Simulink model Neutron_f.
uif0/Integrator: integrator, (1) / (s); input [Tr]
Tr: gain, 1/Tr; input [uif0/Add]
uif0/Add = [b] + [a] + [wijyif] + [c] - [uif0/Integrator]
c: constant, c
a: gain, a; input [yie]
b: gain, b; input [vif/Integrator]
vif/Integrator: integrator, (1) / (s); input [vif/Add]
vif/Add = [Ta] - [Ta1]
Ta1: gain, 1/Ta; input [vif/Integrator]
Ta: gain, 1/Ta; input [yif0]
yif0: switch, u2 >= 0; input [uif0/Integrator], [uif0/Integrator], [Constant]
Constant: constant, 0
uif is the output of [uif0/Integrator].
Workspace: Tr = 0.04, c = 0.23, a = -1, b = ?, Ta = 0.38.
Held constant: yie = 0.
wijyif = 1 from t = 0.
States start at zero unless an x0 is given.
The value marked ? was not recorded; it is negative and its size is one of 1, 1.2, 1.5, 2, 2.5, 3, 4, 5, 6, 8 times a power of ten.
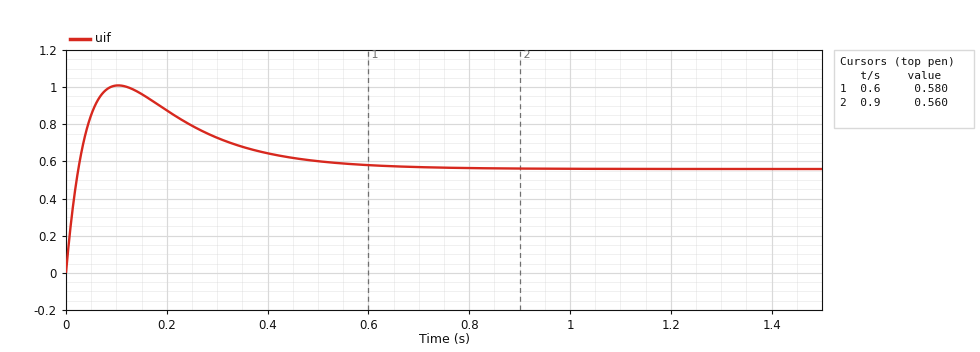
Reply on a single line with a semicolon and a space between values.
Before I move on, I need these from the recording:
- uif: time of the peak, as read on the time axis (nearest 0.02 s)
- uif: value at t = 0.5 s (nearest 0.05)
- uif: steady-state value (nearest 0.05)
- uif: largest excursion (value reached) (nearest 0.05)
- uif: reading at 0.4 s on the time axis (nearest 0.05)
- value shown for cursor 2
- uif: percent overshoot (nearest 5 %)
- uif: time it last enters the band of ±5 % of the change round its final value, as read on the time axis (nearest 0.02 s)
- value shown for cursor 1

0.10 s; 0.60; 0.55; 1.00; 0.65; 0.560; 80 %; 0.56 s; 0.580
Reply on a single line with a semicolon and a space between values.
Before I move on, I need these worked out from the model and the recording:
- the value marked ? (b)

-1.2
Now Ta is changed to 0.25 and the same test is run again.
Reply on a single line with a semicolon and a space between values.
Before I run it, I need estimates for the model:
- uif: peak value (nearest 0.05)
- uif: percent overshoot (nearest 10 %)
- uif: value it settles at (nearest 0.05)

0.95; 70 %; 0.55
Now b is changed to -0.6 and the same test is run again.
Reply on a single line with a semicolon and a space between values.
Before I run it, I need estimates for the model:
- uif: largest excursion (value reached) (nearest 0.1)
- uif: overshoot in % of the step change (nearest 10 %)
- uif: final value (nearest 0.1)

1.1; 40 %; 0.8
